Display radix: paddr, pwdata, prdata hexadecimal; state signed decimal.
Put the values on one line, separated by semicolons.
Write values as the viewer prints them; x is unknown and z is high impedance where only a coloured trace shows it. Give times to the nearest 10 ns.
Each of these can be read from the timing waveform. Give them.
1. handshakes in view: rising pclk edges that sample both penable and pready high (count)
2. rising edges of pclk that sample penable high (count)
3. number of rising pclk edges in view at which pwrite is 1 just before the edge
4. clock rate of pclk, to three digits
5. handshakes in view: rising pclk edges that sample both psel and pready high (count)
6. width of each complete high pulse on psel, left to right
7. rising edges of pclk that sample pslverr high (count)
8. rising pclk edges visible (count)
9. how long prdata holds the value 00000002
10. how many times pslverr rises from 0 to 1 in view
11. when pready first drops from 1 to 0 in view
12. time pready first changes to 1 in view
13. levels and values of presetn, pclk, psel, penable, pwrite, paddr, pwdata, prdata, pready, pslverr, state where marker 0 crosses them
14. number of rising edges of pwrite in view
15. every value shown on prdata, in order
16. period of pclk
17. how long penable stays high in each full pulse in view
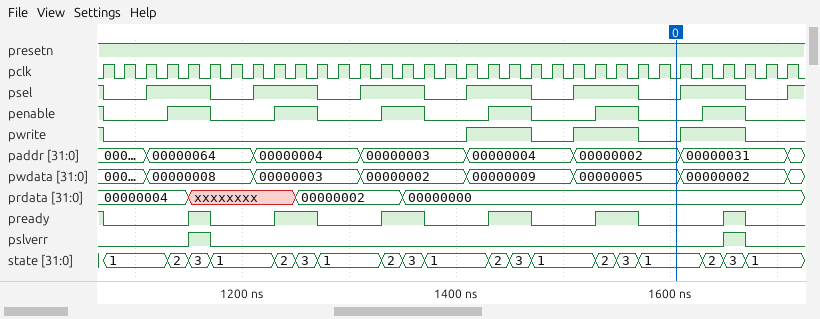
11; 13; 10; 50.0 MHz; 11; 60 ns, 60 ns, 60 ns, 60 ns, 60 ns, 60 ns; 2; 33; 100 ns; 2; 1070 ns; 1150 ns; presetn=1, pclk=0, psel=0, penable=0, pwrite=0, paddr=00000002, pwdata=00000005, prdata=00000000, pready=0, pslverr=0, state=1; 3; 00000004, xxxxxxxx, 00000002, 00000000; 20 ns; 40 ns, 40 ns, 40 ns, 40 ns, 40 ns, 40 ns
